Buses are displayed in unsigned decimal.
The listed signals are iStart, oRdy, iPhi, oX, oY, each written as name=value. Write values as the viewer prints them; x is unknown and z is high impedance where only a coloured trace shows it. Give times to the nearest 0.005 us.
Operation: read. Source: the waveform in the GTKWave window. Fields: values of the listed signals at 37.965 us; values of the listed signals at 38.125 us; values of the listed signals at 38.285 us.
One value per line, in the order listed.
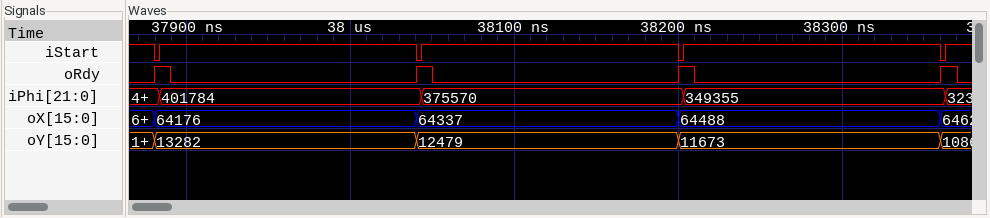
iStart=1, oRdy=0, iPhi=401784, oX=64176, oY=13282
iStart=1, oRdy=0, iPhi=375570, oX=64337, oY=12479
iStart=1, oRdy=0, iPhi=349355, oX=64488, oY=11673
